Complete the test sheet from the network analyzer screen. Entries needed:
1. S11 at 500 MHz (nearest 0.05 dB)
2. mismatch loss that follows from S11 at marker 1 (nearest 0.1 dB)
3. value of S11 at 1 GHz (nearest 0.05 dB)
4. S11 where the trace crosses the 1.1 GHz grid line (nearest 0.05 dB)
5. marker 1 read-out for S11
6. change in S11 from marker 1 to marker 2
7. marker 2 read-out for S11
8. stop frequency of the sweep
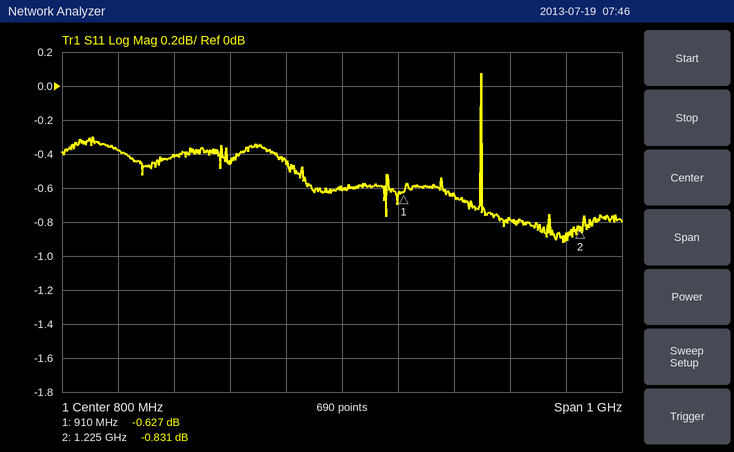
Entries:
-0.40 dB
8.7 dB
-0.65 dB
-0.80 dB
-0.627 dB
-0.204 dB
-0.831 dB
1.3 GHz
